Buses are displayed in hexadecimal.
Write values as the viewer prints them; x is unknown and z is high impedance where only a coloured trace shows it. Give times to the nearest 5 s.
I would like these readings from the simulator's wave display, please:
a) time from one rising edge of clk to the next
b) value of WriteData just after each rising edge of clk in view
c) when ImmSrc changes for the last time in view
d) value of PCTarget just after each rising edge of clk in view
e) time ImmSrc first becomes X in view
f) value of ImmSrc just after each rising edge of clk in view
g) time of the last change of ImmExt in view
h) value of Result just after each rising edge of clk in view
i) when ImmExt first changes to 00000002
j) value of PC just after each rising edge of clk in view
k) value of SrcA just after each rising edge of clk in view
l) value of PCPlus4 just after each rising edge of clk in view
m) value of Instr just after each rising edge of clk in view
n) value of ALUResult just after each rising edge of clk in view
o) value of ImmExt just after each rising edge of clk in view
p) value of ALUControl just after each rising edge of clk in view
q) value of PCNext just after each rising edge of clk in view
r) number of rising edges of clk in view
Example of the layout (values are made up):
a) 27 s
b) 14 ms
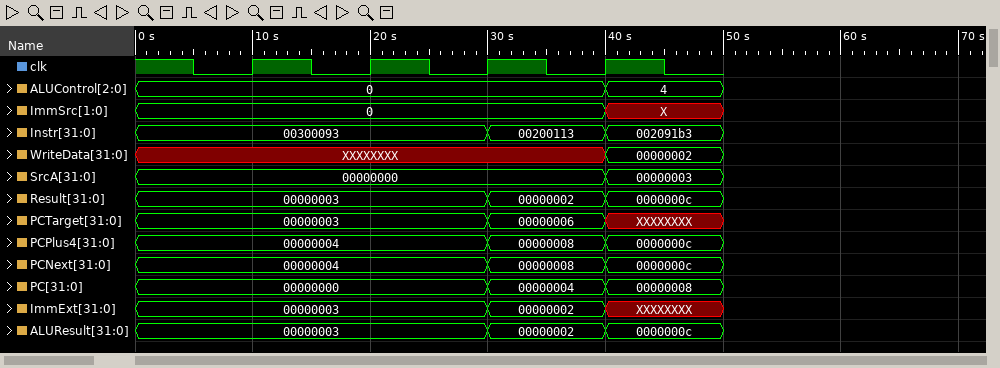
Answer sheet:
a) 10 s
b) XXXXXXXX, XXXXXXXX, XXXXXXXX, 00000002
c) 40 s
d) 00000003, 00000003, 00000006, XXXXXXXX
e) 40 s
f) 0, 0, 0, X
g) 40 s
h) 00000003, 00000003, 00000002, 0000000c
i) 30 s
j) 00000000, 00000000, 00000004, 00000008
k) 00000000, 00000000, 00000000, 00000003
l) 00000004, 00000004, 00000008, 0000000c
m) 00300093, 00300093, 00200113, 002091b3
n) 00000003, 00000003, 00000002, 0000000c
o) 00000003, 00000003, 00000002, XXXXXXXX
p) 0, 0, 0, 4
q) 00000004, 00000004, 00000008, 0000000c
r) 4
